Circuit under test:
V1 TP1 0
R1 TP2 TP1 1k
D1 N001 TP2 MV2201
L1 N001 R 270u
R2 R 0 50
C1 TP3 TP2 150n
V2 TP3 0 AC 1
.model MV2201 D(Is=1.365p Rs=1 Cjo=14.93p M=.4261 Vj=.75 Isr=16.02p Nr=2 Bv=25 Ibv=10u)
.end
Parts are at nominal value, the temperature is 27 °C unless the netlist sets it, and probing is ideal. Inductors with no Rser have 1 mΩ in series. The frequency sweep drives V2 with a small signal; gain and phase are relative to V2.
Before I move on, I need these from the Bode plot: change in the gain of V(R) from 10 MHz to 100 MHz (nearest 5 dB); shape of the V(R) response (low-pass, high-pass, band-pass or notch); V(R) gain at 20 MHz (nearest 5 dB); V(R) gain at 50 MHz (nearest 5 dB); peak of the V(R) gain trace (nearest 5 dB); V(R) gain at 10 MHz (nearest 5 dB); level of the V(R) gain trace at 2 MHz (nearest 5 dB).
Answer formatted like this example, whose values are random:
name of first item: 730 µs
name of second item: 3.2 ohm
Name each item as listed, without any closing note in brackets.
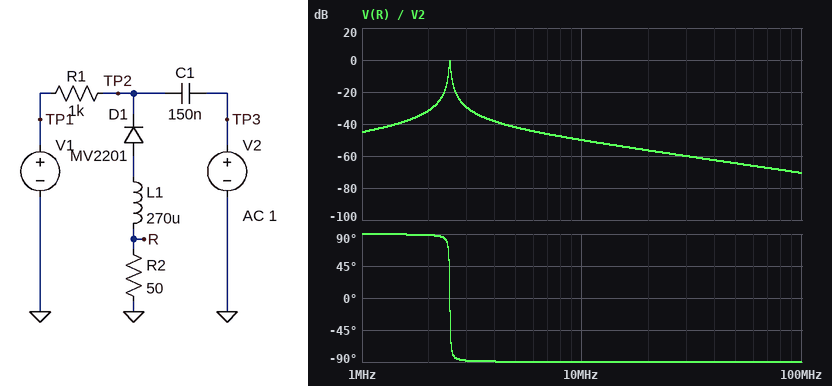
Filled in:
change in the gain of V(R) from 10 MHz to 100 MHz: -20 dB
shape of the V(R) response: band-pass
V(R) gain at 20 MHz: -55 dB
V(R) gain at 50 MHz: -65 dB
peak of the V(R) gain trace: 0 dB
V(R) gain at 10 MHz: -50 dB
level of the V(R) gain trace at 2 MHz: -30 dB
